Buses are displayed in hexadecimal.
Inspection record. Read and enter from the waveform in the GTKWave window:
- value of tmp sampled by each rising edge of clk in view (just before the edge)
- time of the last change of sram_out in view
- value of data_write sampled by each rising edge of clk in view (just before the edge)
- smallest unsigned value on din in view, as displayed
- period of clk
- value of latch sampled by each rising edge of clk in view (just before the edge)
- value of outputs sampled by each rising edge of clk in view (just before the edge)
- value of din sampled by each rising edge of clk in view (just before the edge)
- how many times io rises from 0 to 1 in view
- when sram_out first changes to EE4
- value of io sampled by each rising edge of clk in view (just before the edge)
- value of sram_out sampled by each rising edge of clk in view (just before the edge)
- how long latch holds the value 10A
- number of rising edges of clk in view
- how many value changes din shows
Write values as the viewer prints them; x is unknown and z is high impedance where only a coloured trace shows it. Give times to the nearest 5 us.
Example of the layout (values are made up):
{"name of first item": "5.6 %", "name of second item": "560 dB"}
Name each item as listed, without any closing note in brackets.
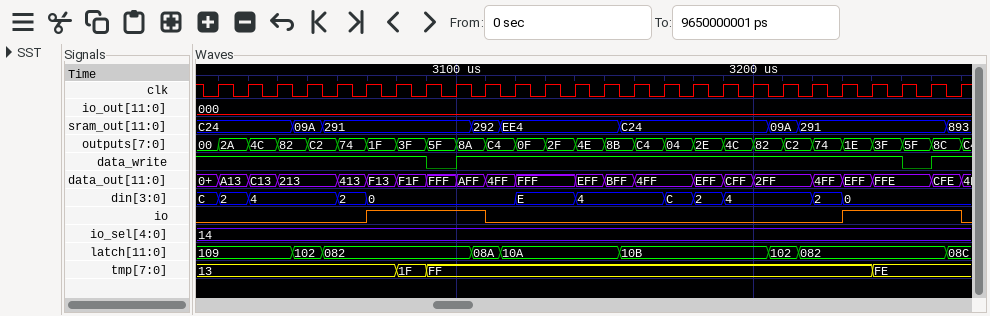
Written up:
{"value of tmp sampled by each rising edge of clk in view": "13, 13, 13, 13, 13, 13, 13, 1F, FF, FF, FF, FF, FF, FF, FF, FF, FF, FF, FF, FF, FF, FF, FF, FE, FE, FE", "time of the last change of sram_out in view": "3265 us", "value of data_write sampled by each rising edge of clk in view": "1 1 1 1 1 1 1 1 0 1 1 1 1 1 1 1 1 1 1 1 1 1 1 1 0 1", "smallest unsigned value on din in view, as displayed": "0", "period of clk": "10 us", "value of latch sampled by each rising edge of clk in view": "109, 109, 109, 102, 082, 082, 082, 082, 082, 08A, 10A, 10A, 10A, 10A, 10B, 10B, 10B, 10B, 10B, 102, 082, 082, 082, 082, 082, 08C", "value of outputs sampled by each rising edge of clk in view": "00, 2A, 4C, 82, C2, 74, 1F, 3F, 5F, 8A, C4, 0F, 2F, 4E, 8B, C4, 04, 2E, 4C, 82, C2, 74, 1E, 3F, 5F, 8C", "value of din sampled by each rising edge of clk in view": "C, 2, 4, 4, 4, 2, 0, 0, 0, 0, 0, E, E, 4, 4, 4, C, 2, 4, 4, 4, 2, 0, 0, 0, 0", "how many times io rises from 0 to 1 in view": "2", "when sram_out first changes to EE4": "3115 us", "value of io sampled by each rising edge of clk in view": "0 0 0 0 0 0 1 1 1 1 0 0 0 0 0 0 0 0 0 0 0 0 1 1 1 1", "value of sram_out sampled by each rising edge of clk in view": "C24, C24, C24, 09A, 291, 291, 291, 291, 291, 292, EE4, EE4, EE4, EE4, C24, C24, C24, C24, C24, 09A, 291, 291, 291, 291, 291, 893", "how long latch holds the value 10A": "40 us", "number of rising edges of clk in view": "26", "how many value changes din shows": "11"}
